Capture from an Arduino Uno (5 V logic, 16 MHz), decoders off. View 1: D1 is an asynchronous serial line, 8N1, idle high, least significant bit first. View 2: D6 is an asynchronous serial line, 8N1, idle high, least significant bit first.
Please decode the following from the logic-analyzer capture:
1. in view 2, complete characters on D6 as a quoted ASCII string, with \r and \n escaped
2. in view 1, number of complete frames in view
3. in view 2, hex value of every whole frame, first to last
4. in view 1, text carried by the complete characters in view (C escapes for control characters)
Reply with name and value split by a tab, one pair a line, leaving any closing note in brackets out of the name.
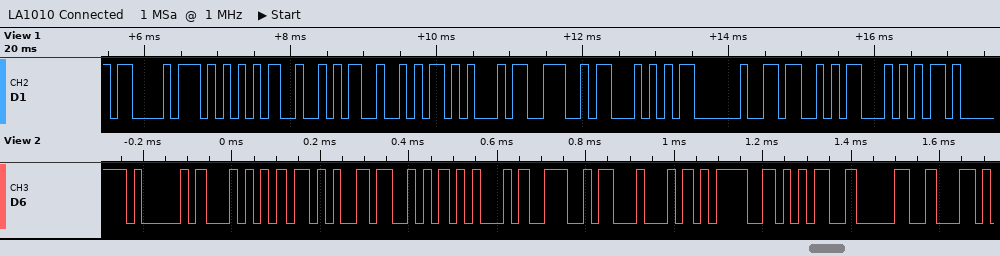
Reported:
in view 2, complete characters on D6 as a quoted ASCII string, with \r and \n escaped	"AT+SEND=50"
in view 1, number of complete frames in view	10
in view 2, hex value of every whole frame, first to last	41 54 2B 53 45 4E 44 3D 35 30
in view 1, text carried by the complete characters in view	"CURRENT ST"
